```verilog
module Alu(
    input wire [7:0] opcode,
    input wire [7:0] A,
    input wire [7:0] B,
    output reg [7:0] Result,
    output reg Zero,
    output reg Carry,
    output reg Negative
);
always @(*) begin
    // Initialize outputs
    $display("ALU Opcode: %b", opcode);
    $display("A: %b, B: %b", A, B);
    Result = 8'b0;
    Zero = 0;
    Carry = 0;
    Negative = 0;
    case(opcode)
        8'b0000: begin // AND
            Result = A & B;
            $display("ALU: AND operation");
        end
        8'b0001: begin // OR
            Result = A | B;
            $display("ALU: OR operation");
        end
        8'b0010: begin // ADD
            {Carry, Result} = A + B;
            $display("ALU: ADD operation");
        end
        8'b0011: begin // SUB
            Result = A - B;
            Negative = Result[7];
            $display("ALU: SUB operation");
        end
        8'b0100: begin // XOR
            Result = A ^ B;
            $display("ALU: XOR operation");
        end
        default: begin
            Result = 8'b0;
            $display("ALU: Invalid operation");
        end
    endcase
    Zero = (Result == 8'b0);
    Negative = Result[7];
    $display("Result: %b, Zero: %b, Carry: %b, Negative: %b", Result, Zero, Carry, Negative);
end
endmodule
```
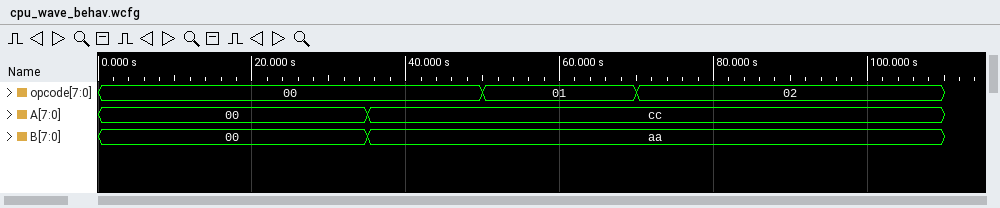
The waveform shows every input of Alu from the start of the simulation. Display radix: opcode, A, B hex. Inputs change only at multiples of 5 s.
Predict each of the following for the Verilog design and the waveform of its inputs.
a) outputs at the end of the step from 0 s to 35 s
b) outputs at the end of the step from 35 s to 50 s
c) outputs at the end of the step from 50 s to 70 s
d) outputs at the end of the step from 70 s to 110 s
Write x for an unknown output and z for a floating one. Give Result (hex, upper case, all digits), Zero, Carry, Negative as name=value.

Result=00, Zero=1, Carry=0, Negative=0
Result=88, Zero=0, Carry=0, Negative=1
Result=EE, Zero=0, Carry=0, Negative=1
Result=76, Zero=0, Carry=1, Negative=0
